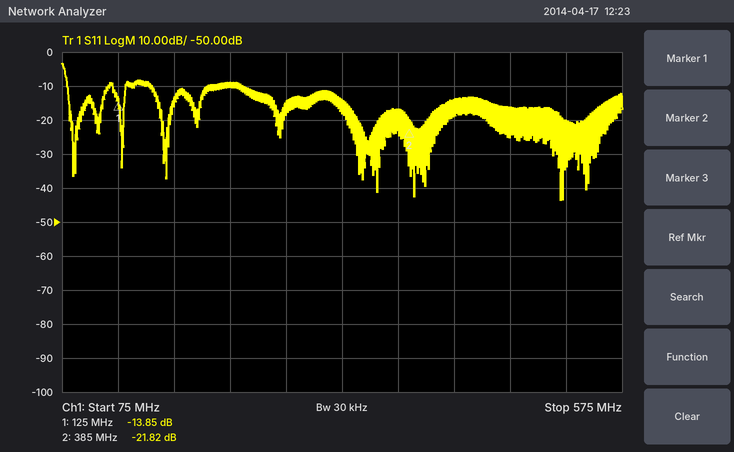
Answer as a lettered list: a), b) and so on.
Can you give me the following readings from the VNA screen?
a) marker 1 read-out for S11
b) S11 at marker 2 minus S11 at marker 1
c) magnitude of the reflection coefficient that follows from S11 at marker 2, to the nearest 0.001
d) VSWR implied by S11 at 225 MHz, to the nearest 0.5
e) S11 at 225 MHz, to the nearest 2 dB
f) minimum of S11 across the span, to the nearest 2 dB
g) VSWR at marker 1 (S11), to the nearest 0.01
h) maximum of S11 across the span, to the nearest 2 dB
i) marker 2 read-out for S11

a) -13.85 dB
b) -7.97 dB
c) 0.081
d) 2.0
e) -10 dB
f) -44 dB
g) 1.51
h) -4 dB
i) -21.82 dB
